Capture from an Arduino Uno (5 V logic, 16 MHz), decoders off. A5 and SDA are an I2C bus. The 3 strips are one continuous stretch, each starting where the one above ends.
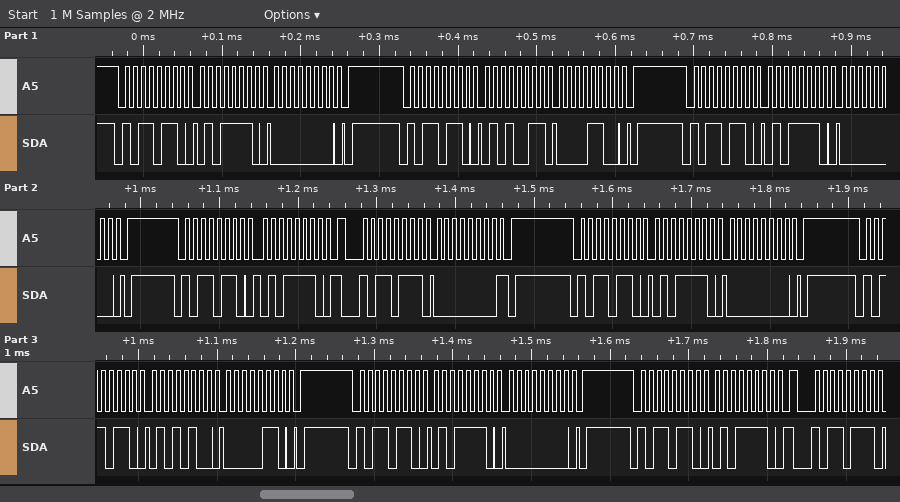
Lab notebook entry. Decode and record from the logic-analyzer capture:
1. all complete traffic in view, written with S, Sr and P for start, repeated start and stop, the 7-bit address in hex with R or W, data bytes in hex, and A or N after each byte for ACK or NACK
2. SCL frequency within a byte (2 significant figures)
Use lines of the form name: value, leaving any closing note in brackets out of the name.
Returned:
all complete traffic in view, written with S, Sr and P for start, repeated start and stop, the 7-bit address in hex with R or W, data bytes in hex, and A or N after each byte for ACK or NACK: S 5BW A 5E A 00 A P S 5BW A 53 A 0C A P S 5BW A 5E A 00 A P S 5BW A 5E A Sr 5BR A 00 N P S 5BW A 5E A 00 A P S 5BW A 54 A 06 A P S 5BW A 5E A 00 A P S 5BW A 5E A Sr 5BR A
SCL frequency within a byte: 100 kHz
